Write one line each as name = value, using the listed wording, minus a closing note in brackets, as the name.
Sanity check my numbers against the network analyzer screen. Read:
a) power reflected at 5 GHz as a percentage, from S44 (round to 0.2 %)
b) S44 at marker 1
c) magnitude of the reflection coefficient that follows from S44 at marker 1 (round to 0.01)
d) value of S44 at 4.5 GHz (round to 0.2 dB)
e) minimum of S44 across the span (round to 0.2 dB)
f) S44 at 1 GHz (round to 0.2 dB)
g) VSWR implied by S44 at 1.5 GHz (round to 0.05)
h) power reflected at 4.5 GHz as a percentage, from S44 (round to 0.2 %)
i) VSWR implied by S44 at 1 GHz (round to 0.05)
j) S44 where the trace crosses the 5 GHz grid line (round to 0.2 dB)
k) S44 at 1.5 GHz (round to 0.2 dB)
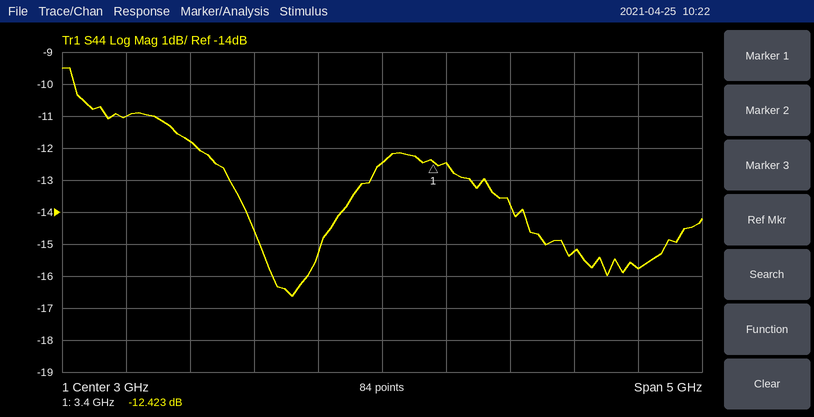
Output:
power reflected at 5 GHz as a percentage, from S44 = 2.6 %
S44 at marker 1 = -12.423 dB
magnitude of the reflection coefficient that follows from S44 at marker 1 = 0.24
value of S44 at 4.5 GHz = -15.2 dB
minimum of S44 across the span = -16.6 dB
S44 at 1 GHz = -11.0 dB
VSWR implied by S44 at 1.5 GHz = 1.70
power reflected at 4.5 GHz as a percentage, from S44 = 3.0 %
VSWR implied by S44 at 1 GHz = 1.80
S44 where the trace crosses the 5 GHz grid line = -15.8 dB
S44 at 1.5 GHz = -11.8 dB
